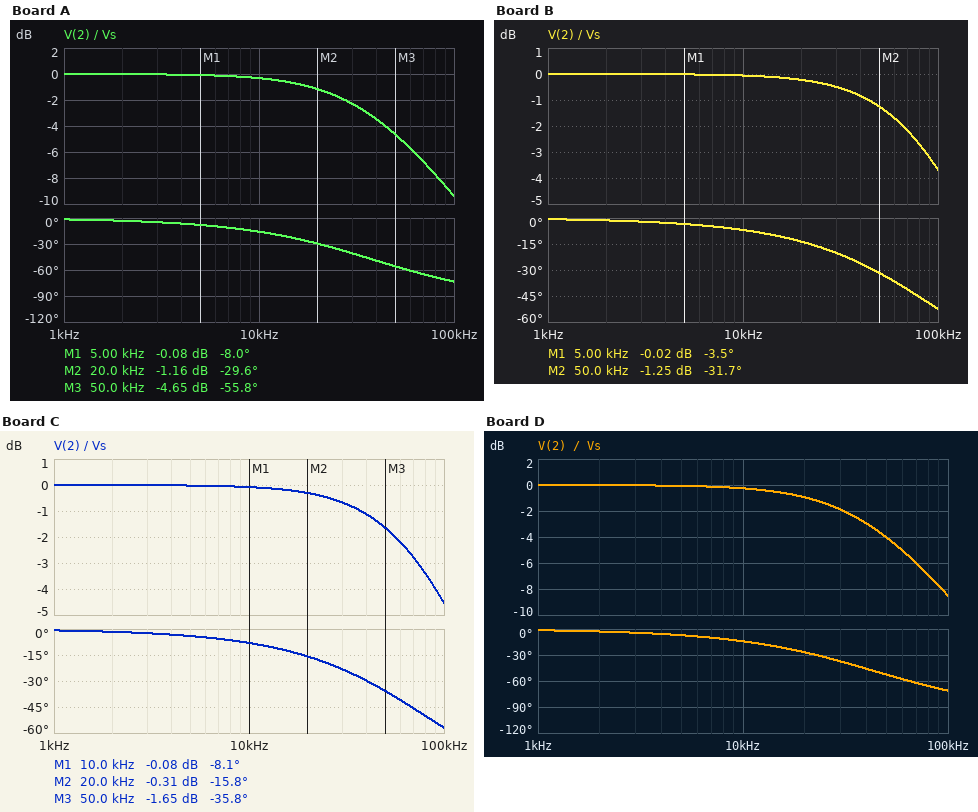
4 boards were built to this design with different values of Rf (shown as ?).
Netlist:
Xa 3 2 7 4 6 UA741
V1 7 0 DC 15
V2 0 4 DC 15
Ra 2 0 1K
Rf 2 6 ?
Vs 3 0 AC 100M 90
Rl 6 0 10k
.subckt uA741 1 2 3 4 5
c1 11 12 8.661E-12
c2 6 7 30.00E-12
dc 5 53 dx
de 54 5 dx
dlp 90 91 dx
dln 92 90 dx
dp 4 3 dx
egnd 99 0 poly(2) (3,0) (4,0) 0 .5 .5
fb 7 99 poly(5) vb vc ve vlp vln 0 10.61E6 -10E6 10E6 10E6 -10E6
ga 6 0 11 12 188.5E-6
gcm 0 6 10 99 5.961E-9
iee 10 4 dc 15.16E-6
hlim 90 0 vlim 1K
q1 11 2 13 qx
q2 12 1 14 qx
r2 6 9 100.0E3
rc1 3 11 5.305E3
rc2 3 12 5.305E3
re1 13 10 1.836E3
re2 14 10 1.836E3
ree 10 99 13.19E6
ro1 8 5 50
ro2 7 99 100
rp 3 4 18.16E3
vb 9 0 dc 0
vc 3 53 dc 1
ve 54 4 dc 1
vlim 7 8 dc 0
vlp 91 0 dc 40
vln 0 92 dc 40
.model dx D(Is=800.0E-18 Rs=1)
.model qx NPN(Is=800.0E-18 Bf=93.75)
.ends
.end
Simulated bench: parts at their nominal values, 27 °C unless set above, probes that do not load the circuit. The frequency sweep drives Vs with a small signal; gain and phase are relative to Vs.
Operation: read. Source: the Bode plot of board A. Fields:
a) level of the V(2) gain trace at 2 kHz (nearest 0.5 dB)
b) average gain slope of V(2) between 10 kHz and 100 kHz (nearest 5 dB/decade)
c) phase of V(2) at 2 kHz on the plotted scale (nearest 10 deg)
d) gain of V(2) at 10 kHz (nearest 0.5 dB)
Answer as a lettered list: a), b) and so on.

a) 0 dB
b) -10 dB/decade
c) 0 deg
d) -0.5 dB
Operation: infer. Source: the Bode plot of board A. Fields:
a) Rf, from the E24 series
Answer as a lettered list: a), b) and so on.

a) 27 kΩ
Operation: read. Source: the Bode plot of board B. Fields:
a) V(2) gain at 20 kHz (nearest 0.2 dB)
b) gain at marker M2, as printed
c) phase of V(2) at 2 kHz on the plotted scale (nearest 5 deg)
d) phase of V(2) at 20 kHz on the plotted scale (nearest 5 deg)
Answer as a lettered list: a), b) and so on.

a) -0.2 dB
b) -1.25 dB
c) 0 deg
d) -15 deg
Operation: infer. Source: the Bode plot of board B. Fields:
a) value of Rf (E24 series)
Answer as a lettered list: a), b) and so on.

a) 11 kΩ
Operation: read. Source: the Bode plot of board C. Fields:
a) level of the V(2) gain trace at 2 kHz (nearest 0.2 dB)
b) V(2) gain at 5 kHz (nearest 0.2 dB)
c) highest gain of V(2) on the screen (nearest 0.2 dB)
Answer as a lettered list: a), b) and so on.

a) 0 dB
b) 0 dB
c) 0 dB
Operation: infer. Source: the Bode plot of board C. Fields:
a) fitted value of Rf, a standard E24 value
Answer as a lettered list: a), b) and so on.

a) 13 kΩ
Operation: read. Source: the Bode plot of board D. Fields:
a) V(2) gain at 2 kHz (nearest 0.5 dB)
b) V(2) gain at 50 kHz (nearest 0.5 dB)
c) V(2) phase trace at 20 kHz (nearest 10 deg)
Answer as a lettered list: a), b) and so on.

a) 0 dB
b) -4.0 dB
c) -30 deg
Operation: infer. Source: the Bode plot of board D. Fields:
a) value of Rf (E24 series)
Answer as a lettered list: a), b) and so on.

a) 24 kΩ
